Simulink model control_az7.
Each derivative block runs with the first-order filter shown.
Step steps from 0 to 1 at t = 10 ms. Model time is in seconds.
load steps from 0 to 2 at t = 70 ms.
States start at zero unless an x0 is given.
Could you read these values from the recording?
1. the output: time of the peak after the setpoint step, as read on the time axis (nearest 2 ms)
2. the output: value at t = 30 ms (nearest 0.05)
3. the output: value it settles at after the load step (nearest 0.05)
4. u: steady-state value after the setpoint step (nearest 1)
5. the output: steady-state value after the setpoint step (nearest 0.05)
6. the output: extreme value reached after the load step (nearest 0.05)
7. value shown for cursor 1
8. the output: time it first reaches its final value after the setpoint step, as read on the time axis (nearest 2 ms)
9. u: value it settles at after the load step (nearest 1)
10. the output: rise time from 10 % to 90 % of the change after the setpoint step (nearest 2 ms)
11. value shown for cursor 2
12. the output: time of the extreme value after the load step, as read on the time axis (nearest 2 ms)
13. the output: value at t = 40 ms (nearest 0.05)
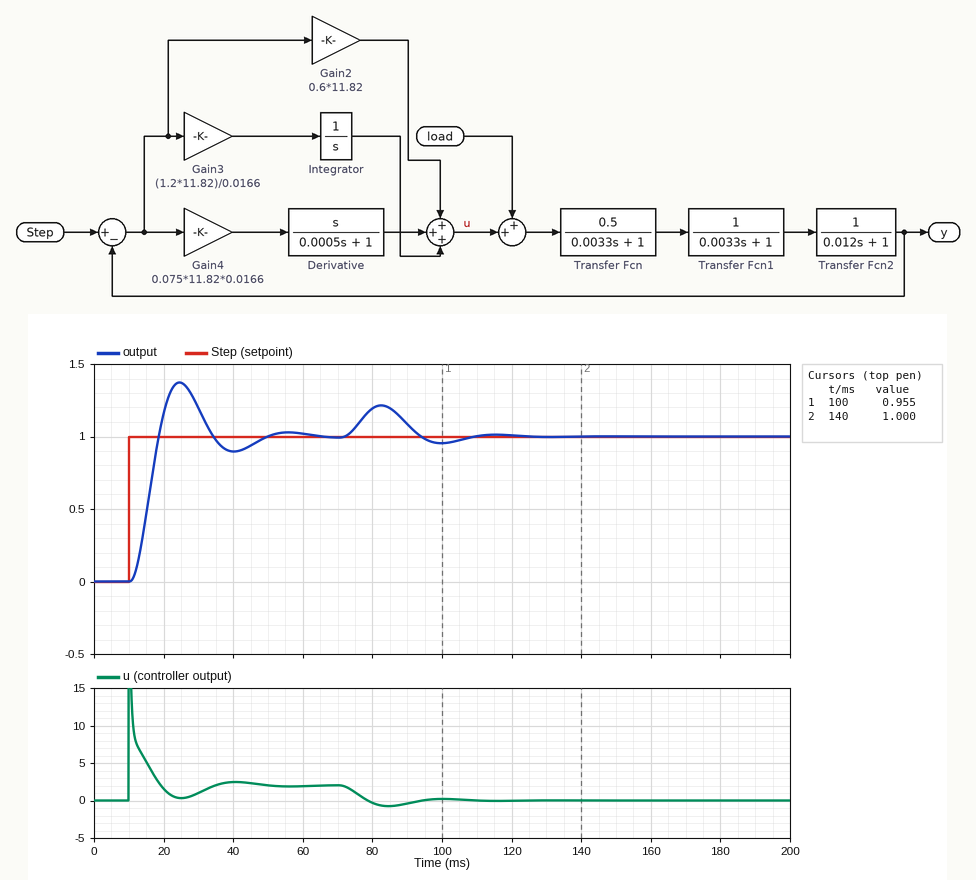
24 ms
1.20
1.00
2
1.00
1.20
0.955
18 ms
0
6 ms
1.000
82 ms
0.90
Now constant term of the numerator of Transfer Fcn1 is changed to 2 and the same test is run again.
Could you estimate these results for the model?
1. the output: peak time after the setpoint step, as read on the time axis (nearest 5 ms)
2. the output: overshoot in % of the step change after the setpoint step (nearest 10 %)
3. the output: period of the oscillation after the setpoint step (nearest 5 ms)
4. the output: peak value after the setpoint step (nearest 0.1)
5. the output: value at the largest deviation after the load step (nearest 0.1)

20 ms
50 %
20 ms
1.5
1.3
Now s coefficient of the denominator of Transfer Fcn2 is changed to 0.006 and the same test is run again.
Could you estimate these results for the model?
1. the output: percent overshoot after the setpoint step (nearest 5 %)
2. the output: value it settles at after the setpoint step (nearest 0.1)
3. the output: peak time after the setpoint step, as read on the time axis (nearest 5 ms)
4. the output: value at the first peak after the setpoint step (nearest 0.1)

30 %
1.0
20 ms
1.3
